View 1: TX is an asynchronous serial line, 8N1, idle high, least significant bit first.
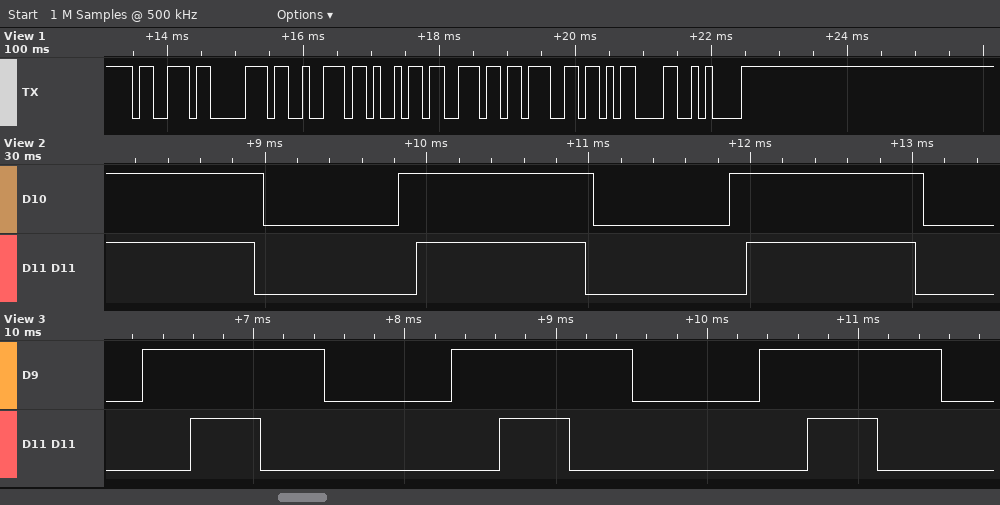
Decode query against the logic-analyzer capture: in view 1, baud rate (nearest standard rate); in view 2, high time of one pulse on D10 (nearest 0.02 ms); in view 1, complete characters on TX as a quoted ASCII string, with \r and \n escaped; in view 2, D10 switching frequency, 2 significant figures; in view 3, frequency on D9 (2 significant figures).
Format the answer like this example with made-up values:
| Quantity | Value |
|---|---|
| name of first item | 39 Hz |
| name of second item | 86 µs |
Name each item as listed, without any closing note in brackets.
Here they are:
| Quantity | Value |
|---|---|
| in view 1, baud rate | 9600 baud |
| in view 2, high time of one pulse on D10 | 1.20 ms |
| in view 1, complete characters on TX as a quoted ASCII string, with \r and \n escaped | "spring\r\n" |
| in view 2, D10 switching frequency, 2 significant figures | 490 Hz |
| in view 3, frequency on D9 | 490 Hz |
